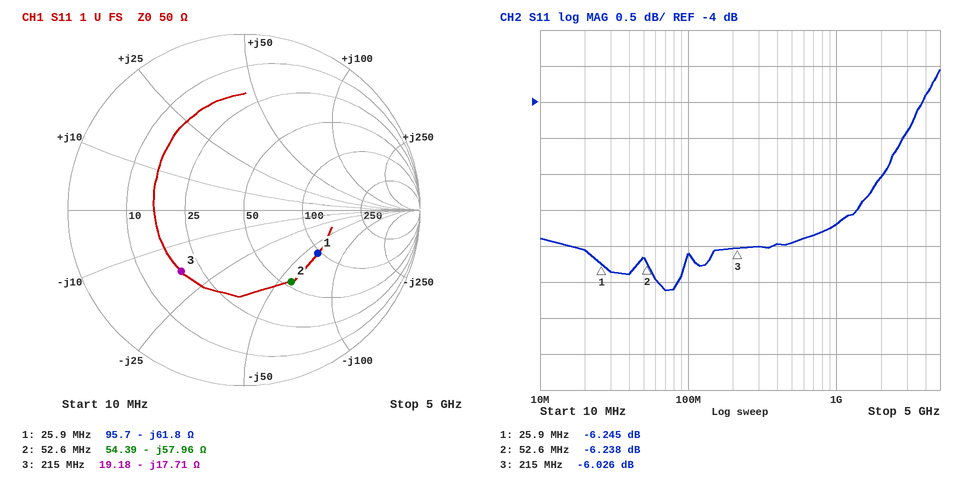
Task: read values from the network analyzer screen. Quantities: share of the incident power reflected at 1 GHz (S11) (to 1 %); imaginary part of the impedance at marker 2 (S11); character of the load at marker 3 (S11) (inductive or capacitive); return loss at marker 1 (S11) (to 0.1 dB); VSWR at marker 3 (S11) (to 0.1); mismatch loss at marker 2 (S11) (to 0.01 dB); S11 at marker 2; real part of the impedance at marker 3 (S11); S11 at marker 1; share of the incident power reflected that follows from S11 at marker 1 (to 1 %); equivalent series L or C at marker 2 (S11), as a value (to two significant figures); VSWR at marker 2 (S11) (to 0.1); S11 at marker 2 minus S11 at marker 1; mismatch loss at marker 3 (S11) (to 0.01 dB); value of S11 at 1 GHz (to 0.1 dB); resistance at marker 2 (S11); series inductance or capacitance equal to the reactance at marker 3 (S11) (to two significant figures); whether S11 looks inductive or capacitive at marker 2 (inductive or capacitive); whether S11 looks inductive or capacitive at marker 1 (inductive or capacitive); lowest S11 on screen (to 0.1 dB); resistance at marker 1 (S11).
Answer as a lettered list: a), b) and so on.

a) 27 %
b) -57.96 Ω
c) capacitive
d) 6.3 dB
e) 3.0
f) 1.18 dB
g) -6.238 dB
h) 19.18 Ω
i) -6.245 dB
j) 24 %
k) 52 pF
l) 2.9
m) 0.007 dB
n) 1.25 dB
o) -5.7 dB
p) 54.39 Ω
q) 42 pF
r) capacitive
s) capacitive
t) -6.6 dB
u) 95.7 Ω
